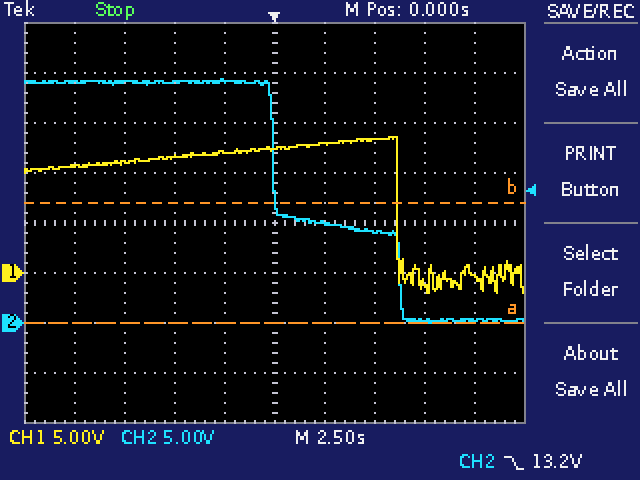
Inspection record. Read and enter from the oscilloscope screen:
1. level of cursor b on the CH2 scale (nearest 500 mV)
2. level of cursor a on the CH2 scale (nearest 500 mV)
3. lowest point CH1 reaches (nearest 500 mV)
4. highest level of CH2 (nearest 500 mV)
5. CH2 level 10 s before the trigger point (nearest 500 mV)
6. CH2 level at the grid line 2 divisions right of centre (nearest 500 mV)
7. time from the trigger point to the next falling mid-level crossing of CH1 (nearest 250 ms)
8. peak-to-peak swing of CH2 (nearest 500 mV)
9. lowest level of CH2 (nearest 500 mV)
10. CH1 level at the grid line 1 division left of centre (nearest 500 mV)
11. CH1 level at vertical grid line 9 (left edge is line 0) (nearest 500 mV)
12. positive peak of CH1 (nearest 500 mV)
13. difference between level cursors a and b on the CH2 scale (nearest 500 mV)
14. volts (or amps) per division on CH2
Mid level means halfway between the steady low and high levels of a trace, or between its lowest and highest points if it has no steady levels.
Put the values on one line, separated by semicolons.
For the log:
12.0 V; 0.0 V; -2.0 V; 24.5 V; 24.0 V; 9.0 V; 6.25 s; 24.5 V; 0.0 V; 12.0 V; -500 mV; 13.5 V; 12.0 V; 5 V
